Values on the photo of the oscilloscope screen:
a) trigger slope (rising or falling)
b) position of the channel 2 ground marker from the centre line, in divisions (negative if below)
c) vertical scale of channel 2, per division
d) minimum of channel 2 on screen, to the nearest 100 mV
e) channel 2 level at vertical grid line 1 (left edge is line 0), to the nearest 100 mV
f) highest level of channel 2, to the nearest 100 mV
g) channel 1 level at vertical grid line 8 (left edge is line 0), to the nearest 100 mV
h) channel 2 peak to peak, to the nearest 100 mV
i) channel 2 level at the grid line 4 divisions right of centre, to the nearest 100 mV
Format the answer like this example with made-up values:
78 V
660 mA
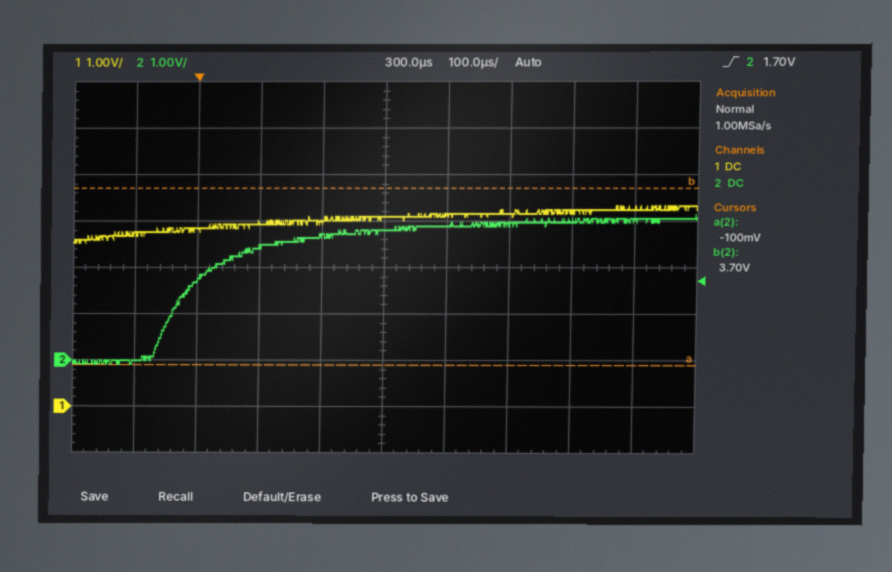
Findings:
rising
-2.0 div
1 V
-100 mV
0.0 V
3.1 V
4.2 V
3.2 V
3.0 V
